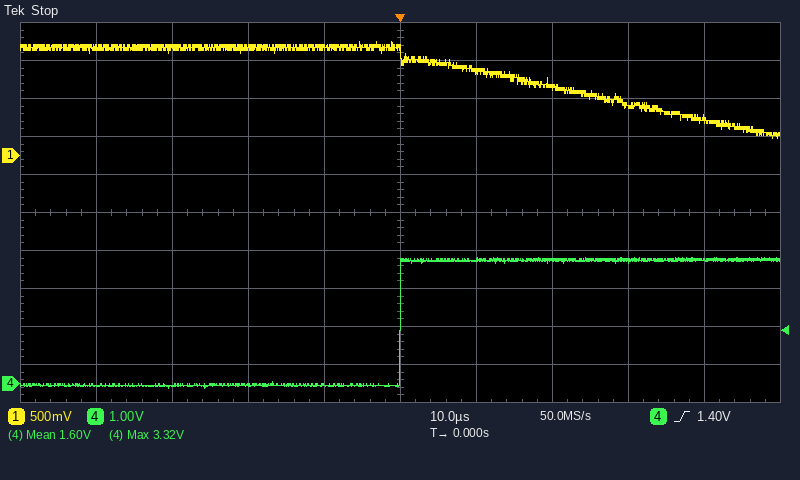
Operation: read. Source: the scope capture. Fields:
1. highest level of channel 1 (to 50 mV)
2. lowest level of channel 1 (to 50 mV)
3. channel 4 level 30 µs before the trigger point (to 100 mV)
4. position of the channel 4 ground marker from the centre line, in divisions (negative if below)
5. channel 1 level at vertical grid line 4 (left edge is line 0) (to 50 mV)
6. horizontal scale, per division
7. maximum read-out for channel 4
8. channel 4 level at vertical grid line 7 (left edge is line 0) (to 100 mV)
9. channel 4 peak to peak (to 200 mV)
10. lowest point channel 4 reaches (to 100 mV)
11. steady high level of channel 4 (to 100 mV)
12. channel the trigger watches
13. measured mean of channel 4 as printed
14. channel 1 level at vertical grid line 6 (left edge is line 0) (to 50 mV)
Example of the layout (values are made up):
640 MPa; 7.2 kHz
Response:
1.50 V; 200 mV; -100 mV; -4.5 div; 1.40 V; 10 µs; 3.32 V; 3.2 V; 3.4 V; -100 mV; 3.2 V; channel 4; 1.60 V; 1.10 V
